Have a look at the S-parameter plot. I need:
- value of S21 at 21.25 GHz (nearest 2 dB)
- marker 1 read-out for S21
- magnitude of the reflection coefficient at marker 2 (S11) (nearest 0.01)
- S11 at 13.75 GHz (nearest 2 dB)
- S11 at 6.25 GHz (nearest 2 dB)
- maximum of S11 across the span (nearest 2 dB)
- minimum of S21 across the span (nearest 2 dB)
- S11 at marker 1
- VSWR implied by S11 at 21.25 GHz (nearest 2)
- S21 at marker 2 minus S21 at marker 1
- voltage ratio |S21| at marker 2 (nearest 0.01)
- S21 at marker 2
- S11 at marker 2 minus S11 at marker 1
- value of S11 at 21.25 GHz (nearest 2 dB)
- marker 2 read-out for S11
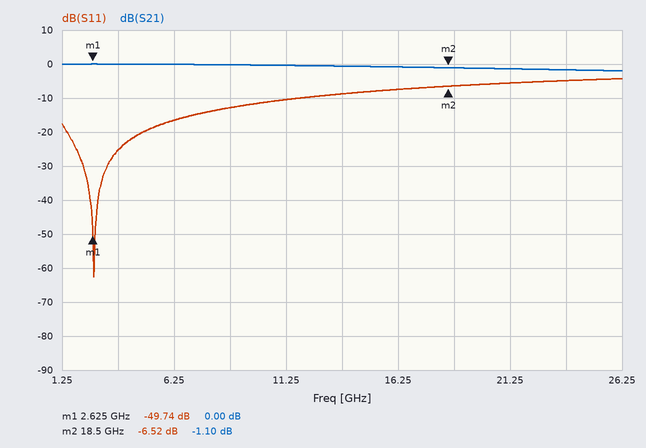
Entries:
-2 dB
0.00 dB
0.47
-8 dB
-16 dB
-4 dB
-2 dB
-49.74 dB
4
-1.10 dB
0.88
-1.10 dB
43.22 dB
-6 dB
-6.52 dB
